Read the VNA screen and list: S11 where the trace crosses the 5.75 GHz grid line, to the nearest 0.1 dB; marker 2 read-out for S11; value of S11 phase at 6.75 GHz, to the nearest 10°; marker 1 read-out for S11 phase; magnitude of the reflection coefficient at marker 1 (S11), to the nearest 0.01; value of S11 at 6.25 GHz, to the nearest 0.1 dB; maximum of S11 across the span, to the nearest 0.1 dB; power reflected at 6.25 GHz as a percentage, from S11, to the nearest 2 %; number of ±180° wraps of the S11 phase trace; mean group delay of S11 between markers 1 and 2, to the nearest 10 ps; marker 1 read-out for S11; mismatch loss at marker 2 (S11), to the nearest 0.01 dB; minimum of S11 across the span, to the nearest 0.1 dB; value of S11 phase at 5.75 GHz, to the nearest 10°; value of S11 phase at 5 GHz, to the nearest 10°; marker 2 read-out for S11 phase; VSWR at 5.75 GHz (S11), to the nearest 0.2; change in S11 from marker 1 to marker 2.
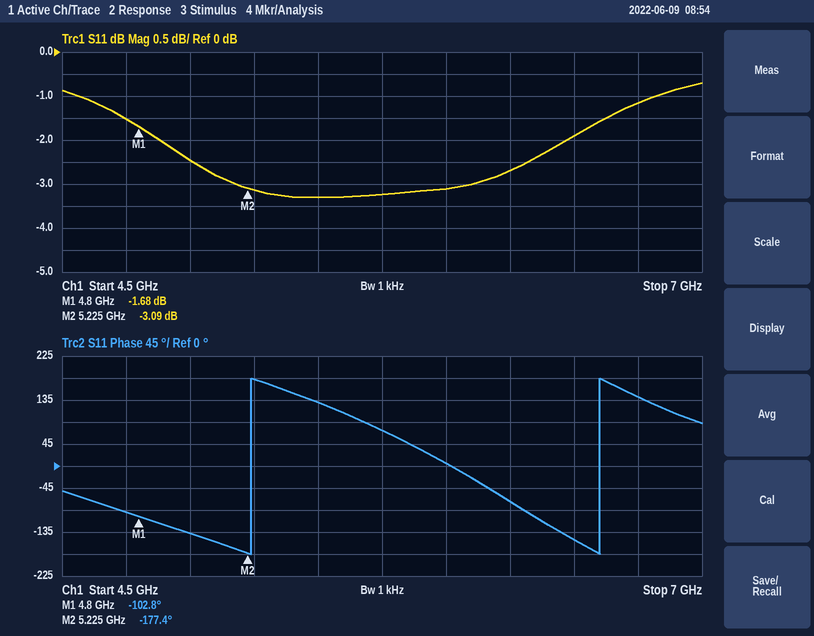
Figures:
-3.2 dB
-3.09 dB
140°
-102.8°
0.82
-2.7 dB
-0.7 dB
54 %
2
490 ps
-1.68 dB
2.93 dB
-3.3 dB
70°
-140°
-177.4°
5.4
-1.41 dB
